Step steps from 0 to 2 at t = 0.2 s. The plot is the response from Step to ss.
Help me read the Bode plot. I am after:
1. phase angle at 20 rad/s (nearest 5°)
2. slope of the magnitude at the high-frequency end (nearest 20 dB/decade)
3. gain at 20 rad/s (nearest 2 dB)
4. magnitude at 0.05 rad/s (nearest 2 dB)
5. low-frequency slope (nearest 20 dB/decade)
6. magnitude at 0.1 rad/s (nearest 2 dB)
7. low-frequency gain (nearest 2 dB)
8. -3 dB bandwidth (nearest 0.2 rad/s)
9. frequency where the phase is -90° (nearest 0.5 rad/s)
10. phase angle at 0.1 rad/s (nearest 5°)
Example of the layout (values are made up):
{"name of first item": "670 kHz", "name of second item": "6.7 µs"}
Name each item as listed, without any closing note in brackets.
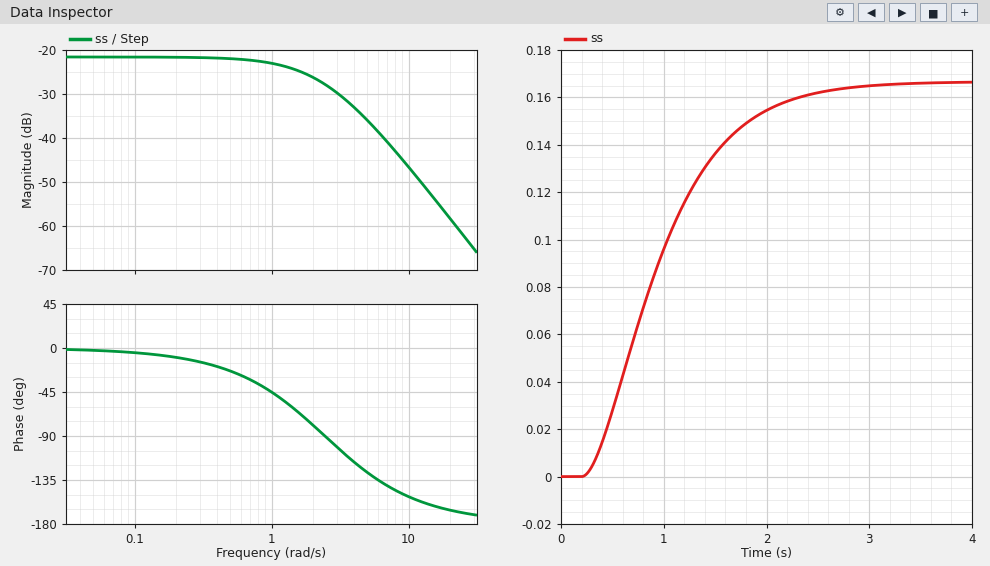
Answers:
{"phase angle at 20 rad/s": "-165°", "slope of the magnitude at the high-frequency end": "-40 dB/decade", "gain at 20 rad/s": "-58 dB", "magnitude at 0.05 rad/s": "-22 dB", "low-frequency slope": "0 dB/decade", "magnitude at 0.1 rad/s": "-22 dB", "low-frequency gain": "-22 dB", "-3 dB bandwidth": "1.6 rad/s", "frequency where the phase is -90°": "2.5 rad/s", "phase angle at 0.1 rad/s": "-5°"}
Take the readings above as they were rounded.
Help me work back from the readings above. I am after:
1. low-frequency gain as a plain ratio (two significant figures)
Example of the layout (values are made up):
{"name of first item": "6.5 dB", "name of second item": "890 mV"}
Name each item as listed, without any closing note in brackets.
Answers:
{"low-frequency gain as a plain ratio": "0.079"}
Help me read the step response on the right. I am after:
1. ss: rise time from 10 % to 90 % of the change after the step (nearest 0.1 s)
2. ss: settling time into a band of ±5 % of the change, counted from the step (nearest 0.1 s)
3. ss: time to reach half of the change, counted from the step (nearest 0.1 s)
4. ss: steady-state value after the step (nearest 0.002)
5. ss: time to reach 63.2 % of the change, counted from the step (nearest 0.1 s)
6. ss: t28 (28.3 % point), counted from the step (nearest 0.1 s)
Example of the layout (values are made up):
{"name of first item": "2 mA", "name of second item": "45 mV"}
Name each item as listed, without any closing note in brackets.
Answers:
{"ss: rise time from 10 % to 90 % of the change after the step": "1.4 s", "ss: settling time into a band of ±5 % of the change, counted from the step": "2.0 s", "ss: time to reach half of the change, counted from the step": "0.7 s", "ss: steady-state value after the step": "0.166", "ss: time to reach 63.2 % of the change, counted from the step": "0.9 s", "ss: t28 (28.3 % point), counted from the step": "0.4 s"}
